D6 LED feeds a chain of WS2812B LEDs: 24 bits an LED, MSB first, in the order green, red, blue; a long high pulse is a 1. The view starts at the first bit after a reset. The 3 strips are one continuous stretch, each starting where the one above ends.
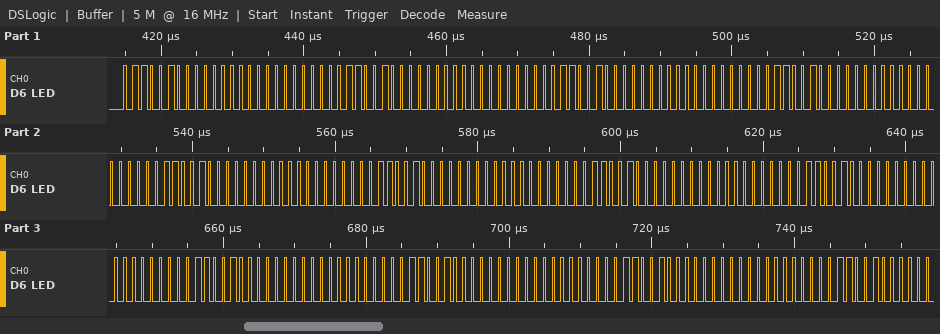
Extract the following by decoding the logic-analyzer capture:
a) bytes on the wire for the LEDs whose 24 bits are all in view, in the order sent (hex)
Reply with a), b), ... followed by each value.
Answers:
a) 64 00 00 64 00 00 64 00 00 64 00 00 64 00 00 64 00 00 64 00 00 64 00 00 64 00 00 64 00 00 64 00 00
